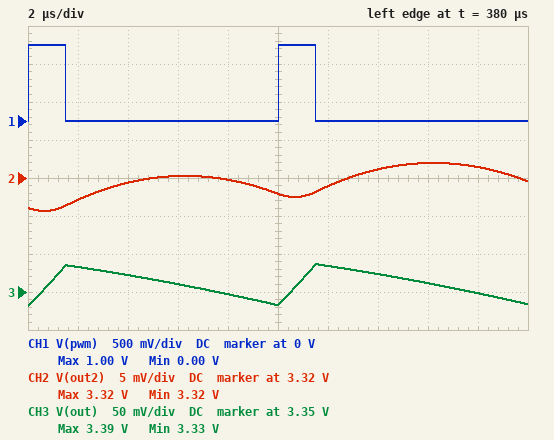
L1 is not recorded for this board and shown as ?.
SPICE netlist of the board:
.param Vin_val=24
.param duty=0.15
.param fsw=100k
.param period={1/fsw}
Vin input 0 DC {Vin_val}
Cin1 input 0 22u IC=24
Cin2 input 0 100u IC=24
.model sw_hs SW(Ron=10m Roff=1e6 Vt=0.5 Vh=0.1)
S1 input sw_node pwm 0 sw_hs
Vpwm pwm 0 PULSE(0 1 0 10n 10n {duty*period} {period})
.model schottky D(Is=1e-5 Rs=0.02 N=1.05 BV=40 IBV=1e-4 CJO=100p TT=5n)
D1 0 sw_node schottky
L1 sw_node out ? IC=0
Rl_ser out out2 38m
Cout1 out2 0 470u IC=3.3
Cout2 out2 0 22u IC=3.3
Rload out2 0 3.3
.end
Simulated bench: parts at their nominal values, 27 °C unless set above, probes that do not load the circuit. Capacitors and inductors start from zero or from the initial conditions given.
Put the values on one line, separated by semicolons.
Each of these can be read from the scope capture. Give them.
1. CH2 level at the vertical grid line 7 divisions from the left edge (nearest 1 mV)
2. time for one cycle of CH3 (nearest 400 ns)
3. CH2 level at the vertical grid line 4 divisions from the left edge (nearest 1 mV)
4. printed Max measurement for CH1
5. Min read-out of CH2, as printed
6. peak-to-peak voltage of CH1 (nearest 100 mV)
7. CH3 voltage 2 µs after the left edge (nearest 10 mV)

3.321 V; 10.0 µs; 3.320 V; 1.00 V; 3.32 V; 1.0 V; 3.38 V
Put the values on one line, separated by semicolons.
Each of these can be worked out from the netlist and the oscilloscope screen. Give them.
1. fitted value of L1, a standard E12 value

22 µH
